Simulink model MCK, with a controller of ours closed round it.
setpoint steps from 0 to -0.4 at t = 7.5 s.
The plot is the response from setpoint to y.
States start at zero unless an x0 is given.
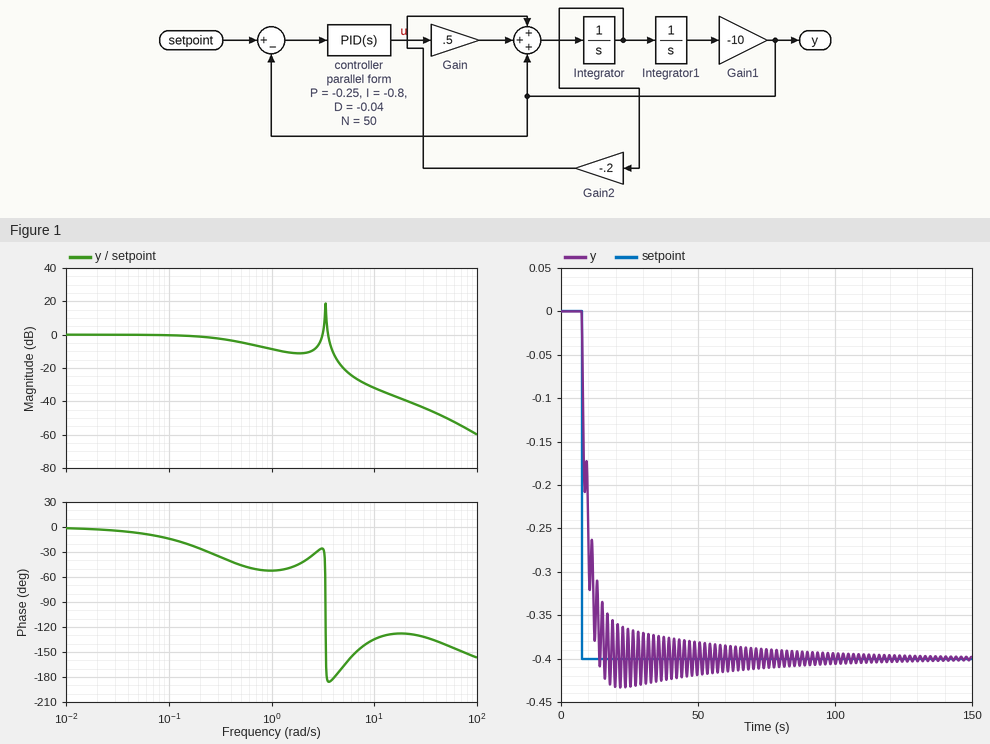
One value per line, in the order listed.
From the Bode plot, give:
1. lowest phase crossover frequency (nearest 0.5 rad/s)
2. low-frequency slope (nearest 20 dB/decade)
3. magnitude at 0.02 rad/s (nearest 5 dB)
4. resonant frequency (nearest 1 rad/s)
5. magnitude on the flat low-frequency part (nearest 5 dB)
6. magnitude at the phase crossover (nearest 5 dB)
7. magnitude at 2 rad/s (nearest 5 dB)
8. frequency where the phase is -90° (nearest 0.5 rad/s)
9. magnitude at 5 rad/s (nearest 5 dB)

3.5 rad/s
0 dB/decade
0 dB
3 rad/s
0 dB
5 dB
-10 dB
3.5 rad/s
-20 dB
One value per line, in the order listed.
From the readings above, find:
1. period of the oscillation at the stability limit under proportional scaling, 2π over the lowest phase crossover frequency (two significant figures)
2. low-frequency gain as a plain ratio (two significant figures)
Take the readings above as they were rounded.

1.8 s
1.0
